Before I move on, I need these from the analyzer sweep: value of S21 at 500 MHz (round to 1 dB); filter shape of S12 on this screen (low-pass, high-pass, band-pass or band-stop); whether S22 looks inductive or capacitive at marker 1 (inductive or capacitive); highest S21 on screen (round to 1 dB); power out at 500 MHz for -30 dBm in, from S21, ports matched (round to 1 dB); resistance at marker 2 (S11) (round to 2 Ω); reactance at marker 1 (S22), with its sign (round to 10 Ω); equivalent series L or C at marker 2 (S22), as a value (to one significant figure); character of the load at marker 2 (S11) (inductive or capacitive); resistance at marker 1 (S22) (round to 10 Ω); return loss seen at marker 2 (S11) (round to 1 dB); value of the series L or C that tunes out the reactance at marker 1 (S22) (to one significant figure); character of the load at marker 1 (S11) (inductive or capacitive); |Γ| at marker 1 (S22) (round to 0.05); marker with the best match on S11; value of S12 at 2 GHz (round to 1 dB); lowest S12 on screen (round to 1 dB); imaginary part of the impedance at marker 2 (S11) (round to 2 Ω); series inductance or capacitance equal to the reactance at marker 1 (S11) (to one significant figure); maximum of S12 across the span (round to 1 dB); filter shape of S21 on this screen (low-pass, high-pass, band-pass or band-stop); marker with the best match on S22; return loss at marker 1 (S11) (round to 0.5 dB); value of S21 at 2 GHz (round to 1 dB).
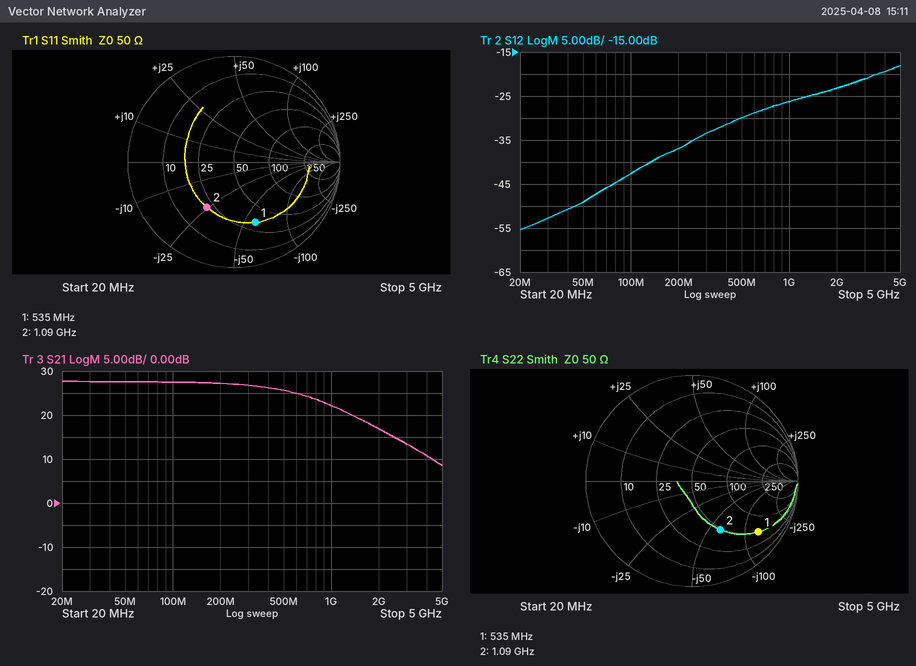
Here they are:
26 dB
high-pass
capacitive
28 dB
-4 dBm
22 Ω
-130 Ω
2 pF
capacitive
50 Ω
6 dB
40 nH
capacitive
0.80
marker 2
-23 dB
-55 dB
-24 Ω
5 pF
-18 dB
low-pass
marker 2
4.5 dB
17 dB
